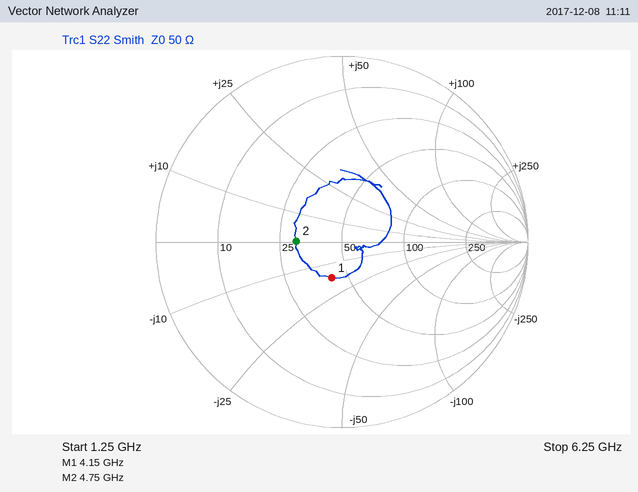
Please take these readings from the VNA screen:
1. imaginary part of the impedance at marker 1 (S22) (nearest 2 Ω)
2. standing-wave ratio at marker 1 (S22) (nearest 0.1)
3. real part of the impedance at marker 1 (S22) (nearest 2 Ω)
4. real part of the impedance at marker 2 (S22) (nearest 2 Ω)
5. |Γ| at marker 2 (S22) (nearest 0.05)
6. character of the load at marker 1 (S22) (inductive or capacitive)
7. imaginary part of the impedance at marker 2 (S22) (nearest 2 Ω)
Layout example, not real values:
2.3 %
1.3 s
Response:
-16 Ω
1.5
42 Ω
30 Ω
0.25
capacitive
0 Ω
